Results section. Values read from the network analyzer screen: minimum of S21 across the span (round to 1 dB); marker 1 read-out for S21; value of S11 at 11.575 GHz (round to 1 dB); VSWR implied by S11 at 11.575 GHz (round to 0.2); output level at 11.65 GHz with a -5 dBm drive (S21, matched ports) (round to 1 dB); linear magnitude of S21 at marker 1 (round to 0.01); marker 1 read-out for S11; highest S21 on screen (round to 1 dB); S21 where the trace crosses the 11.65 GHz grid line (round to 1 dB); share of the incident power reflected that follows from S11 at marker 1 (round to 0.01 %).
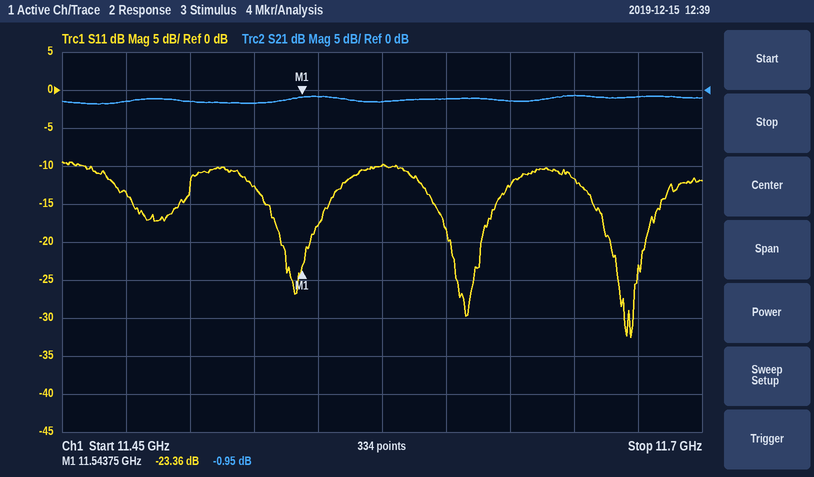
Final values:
-2 dB
-0.95 dB
-10 dB
2.0
-6 dBm
0.90
-23.36 dB
-1 dB
-1 dB
0.46 %
